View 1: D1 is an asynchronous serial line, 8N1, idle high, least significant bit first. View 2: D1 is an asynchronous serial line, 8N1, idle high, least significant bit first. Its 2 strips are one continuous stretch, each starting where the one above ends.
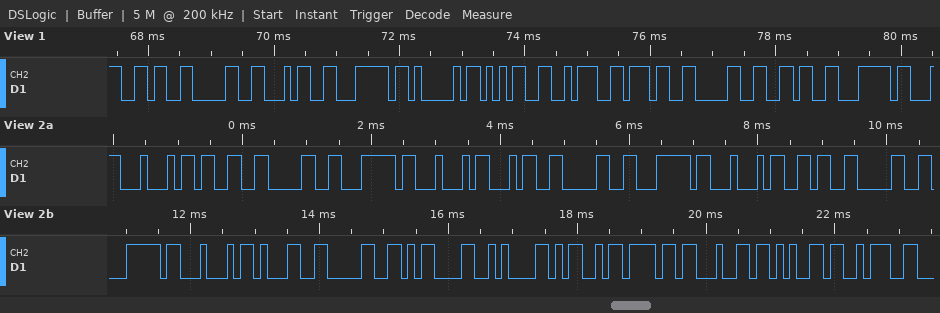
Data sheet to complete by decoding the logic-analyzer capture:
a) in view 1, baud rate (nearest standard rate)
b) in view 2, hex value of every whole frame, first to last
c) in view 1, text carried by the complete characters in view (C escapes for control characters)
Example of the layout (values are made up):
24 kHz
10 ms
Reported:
9600 baud
0x44 0x33 0x30 0x7C 0x44 0x34 0x30 0x7C 0x44 0x36 0x30 0x7C 0x44 0x31 0x30 0x0D 0x0A 0x4D 0x6F 0x64 0x65 0x3A
"604|A5:706|"
